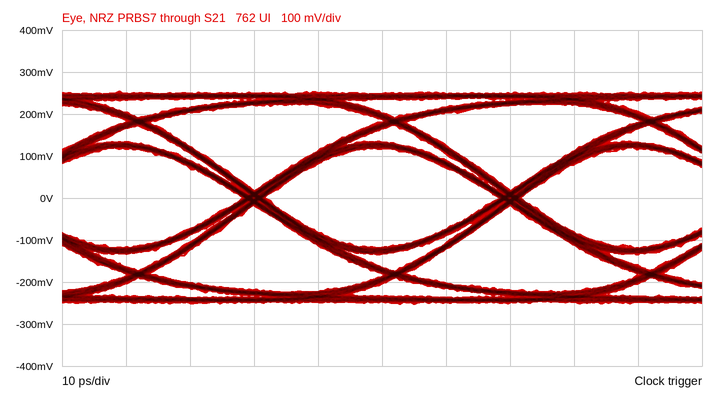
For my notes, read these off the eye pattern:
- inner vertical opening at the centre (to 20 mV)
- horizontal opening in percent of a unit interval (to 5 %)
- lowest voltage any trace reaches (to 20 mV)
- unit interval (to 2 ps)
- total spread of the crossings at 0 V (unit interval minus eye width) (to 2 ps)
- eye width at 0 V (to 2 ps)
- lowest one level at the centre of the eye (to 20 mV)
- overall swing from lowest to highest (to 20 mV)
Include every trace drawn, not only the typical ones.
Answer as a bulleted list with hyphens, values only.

- 240 mV
- 90 %
- -260 mV
- 40 ps
- 4 ps
- 36 ps
- 120 mV
- 500 mV
